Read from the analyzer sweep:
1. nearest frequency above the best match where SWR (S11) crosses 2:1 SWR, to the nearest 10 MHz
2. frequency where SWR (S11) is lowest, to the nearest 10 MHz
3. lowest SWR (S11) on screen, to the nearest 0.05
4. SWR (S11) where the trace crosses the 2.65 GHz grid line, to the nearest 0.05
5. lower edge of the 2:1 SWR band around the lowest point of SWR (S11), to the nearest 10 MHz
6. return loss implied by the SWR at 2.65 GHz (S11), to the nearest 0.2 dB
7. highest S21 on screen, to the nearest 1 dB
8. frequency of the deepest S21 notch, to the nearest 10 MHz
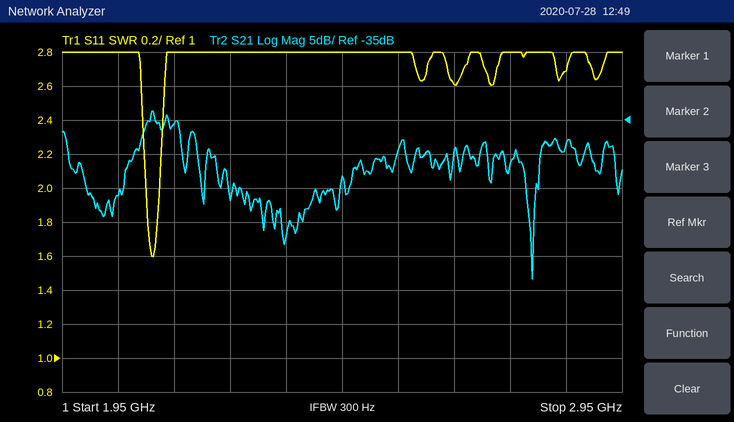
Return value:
2.12 GHz
2.11 GHz
1.60
2.60
2.10 GHz
7.0 dB
-34 dB
2.79 GHz
